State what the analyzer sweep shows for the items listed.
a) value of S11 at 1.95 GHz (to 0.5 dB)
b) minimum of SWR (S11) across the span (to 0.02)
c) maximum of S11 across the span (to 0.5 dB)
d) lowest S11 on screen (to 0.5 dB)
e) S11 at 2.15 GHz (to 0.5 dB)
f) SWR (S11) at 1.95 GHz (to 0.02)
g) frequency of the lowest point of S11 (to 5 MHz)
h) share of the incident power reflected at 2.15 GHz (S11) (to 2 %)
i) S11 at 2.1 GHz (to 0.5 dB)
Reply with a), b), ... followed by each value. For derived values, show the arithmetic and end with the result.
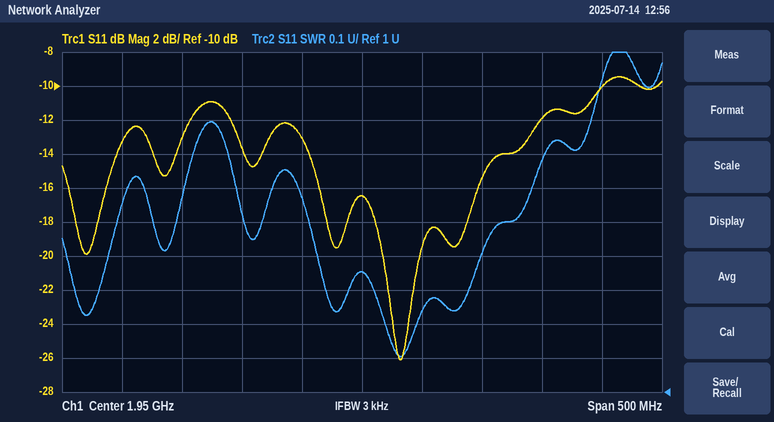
a) -16.5 dB
b) 1.10
c) -9.5 dB
d) -26.0 dB
e) -10.0 dB
f) 1.36
g) 1.980 GHz
h) 10^(-10/10) ≈ 10 %
i) -12.0 dB
